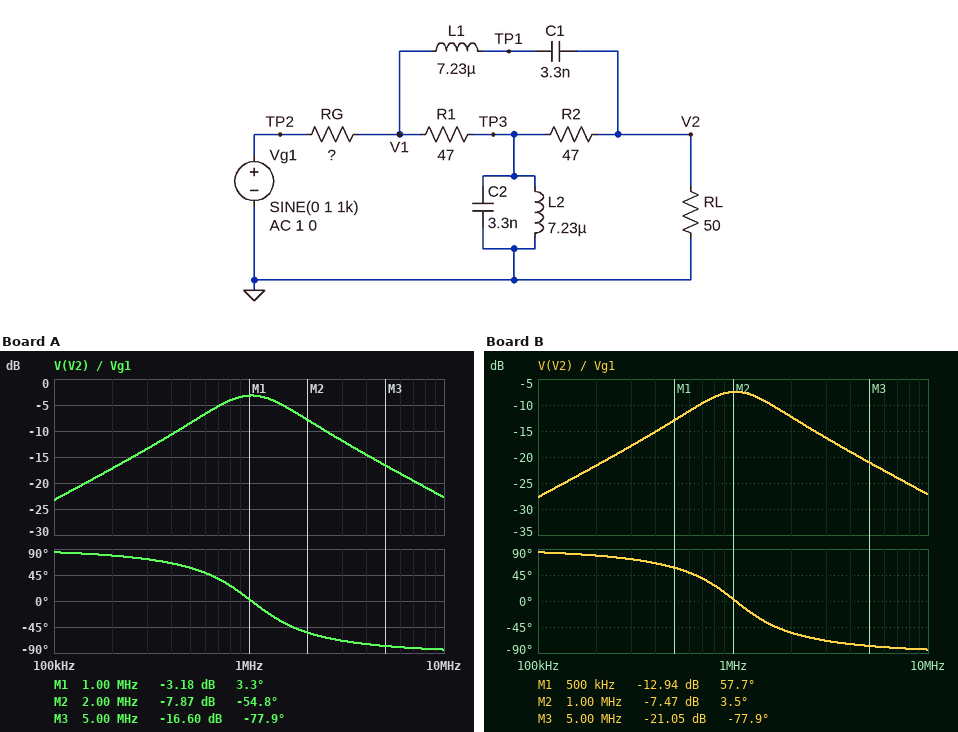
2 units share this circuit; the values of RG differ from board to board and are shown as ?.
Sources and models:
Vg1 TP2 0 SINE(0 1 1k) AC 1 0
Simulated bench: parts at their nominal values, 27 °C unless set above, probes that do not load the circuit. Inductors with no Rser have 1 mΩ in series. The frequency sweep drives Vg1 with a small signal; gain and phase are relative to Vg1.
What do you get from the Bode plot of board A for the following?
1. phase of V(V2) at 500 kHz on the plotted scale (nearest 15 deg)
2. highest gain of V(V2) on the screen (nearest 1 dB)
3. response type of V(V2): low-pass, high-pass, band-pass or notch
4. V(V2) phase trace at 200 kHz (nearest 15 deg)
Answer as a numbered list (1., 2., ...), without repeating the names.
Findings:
1. 60 deg
2. -3 dB
3. band-pass
4. 75 deg
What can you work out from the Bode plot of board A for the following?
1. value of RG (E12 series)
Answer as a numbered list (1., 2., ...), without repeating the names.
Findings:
1. 22 Ω
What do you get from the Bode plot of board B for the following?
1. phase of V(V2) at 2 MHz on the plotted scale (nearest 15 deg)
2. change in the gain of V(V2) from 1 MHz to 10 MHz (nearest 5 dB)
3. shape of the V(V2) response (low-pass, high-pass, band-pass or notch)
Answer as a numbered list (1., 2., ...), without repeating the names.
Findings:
1. -60 deg
2. -20 dB
3. band-pass
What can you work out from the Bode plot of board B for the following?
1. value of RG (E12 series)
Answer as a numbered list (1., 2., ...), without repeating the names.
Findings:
1. 68 Ω
